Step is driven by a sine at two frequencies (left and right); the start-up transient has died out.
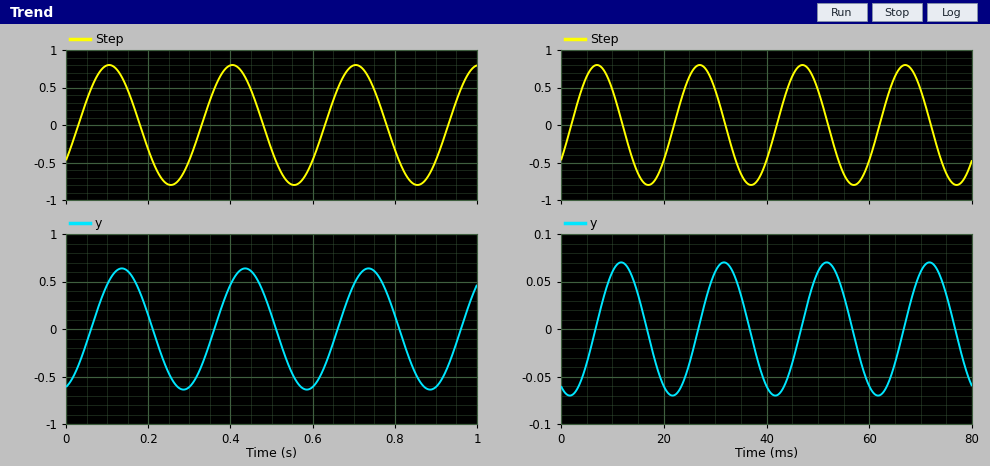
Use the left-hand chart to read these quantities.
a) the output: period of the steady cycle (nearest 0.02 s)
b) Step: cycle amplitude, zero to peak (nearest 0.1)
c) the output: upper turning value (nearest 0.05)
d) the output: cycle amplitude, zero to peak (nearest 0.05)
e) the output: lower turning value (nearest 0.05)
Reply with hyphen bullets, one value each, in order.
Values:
- 0.30 s
- 0.8
- 0.65
- 0.65
- -0.65
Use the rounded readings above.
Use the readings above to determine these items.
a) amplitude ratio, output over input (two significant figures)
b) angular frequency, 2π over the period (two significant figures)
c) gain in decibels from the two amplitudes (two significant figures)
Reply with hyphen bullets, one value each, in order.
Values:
- 0.81
- 21 rad/s
- -1.8 dB
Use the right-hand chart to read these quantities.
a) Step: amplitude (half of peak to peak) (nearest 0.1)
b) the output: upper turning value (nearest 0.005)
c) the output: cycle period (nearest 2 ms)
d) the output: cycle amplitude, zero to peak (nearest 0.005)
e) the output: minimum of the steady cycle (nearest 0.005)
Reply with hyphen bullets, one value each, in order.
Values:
- 0.8
- 0.070
- 20 ms
- 0.070
- -0.070
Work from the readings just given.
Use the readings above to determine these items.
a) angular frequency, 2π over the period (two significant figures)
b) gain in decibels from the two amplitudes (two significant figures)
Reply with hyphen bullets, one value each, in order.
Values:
- 0.31 rad/ms
- -21 dB
